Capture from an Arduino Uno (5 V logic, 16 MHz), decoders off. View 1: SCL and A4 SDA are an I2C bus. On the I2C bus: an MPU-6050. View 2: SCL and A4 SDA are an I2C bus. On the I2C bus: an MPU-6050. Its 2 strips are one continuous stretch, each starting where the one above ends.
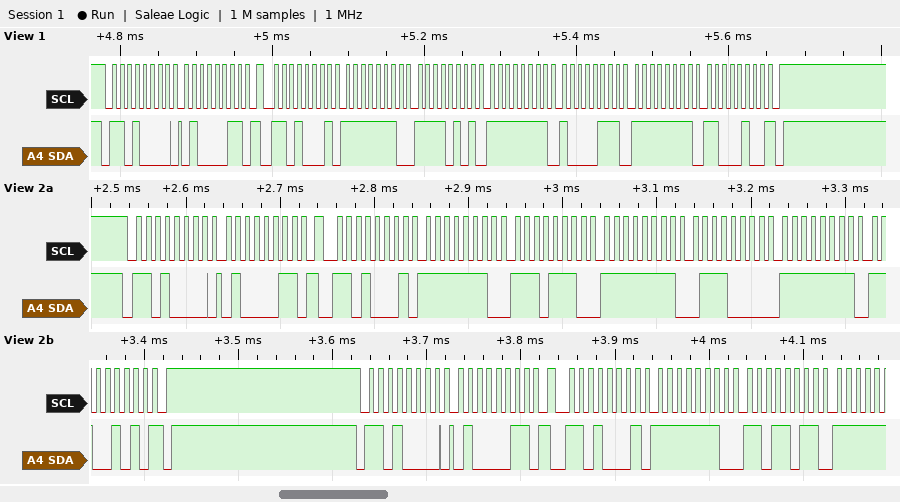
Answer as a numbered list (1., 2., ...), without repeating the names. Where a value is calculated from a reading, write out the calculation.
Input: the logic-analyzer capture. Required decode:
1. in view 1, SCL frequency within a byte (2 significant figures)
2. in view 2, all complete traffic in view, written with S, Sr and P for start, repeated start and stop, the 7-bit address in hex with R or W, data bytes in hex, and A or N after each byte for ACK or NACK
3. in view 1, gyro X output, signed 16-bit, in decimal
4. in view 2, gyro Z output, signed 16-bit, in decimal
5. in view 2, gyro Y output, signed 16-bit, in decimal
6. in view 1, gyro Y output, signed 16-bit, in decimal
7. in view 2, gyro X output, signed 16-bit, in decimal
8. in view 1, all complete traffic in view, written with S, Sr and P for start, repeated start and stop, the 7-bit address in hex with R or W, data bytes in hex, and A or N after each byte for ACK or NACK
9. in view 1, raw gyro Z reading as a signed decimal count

1. 100 kHz
2. S 68W A 43 A Sr 68R A FE A EE A FF A 70 A FF A CA N P S 68W A 43 A Sr 68R A FE A DB A
3. 0xFEF5 = -267
4. 0xFFCA = -54
5. 0xFF70 = -144
6. 0xFF87 = -121
7. 0xFEEE = -274
8. S 68W A 43 A Sr 68R A FE A F5 A FF A 87 A FF A C4 N P
9. 0xFFC4 = -60
